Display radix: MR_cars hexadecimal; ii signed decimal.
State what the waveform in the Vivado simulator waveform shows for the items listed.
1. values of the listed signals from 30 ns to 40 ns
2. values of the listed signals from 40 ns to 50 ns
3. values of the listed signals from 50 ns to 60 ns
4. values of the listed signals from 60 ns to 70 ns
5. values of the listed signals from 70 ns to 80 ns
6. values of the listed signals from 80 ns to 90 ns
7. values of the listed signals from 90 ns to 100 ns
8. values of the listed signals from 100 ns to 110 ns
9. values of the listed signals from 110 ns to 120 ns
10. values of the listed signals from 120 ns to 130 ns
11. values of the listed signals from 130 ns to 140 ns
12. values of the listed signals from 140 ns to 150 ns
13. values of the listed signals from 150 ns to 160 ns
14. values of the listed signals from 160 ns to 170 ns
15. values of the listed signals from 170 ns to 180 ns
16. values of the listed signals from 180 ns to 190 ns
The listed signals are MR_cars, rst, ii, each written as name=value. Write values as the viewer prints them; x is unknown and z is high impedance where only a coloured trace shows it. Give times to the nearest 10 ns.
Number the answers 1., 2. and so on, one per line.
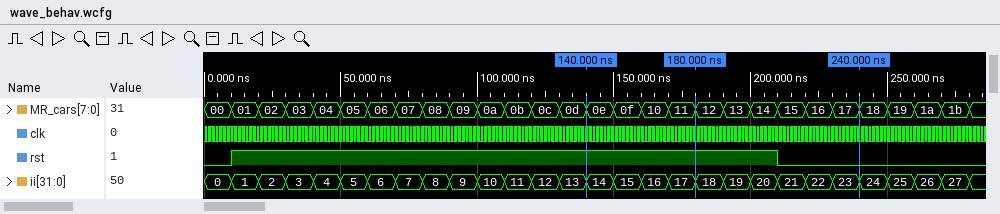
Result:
1. MR_cars=03, rst=1, ii=3
2. MR_cars=04, rst=1, ii=4
3. MR_cars=05, rst=1, ii=5
4. MR_cars=06, rst=1, ii=6
5. MR_cars=07, rst=1, ii=7
6. MR_cars=08, rst=1, ii=8
7. MR_cars=09, rst=1, ii=9
8. MR_cars=0a, rst=1, ii=10
9. MR_cars=0b, rst=1, ii=11
10. MR_cars=0c, rst=1, ii=12
11. MR_cars=0d, rst=1, ii=13
12. MR_cars=0e, rst=1, ii=14
13. MR_cars=0f, rst=1, ii=15
14. MR_cars=10, rst=1, ii=16
15. MR_cars=11, rst=1, ii=17
16. MR_cars=12, rst=1, ii=18
